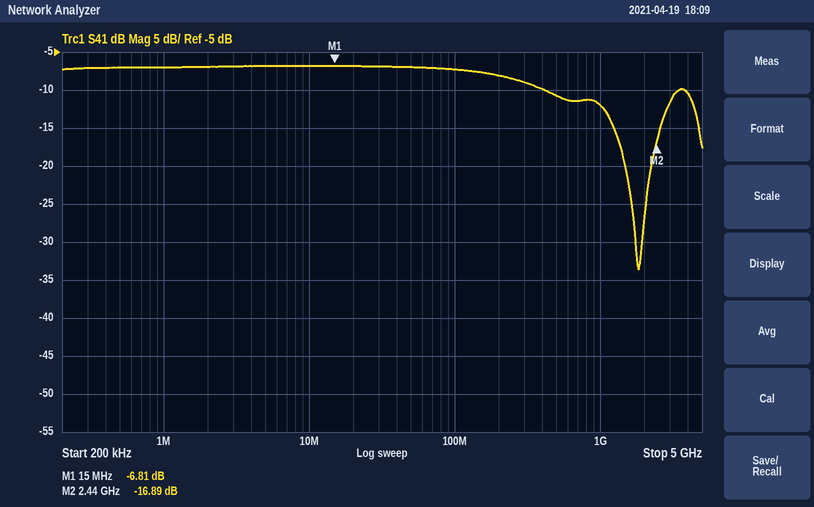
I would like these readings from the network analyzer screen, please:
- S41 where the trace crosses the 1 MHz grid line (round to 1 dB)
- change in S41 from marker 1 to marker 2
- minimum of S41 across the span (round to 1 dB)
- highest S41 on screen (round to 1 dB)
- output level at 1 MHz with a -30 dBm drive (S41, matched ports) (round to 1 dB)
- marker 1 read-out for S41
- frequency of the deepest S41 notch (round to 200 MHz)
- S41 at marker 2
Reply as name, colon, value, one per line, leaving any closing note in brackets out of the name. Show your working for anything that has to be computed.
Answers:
S41 where the trace crosses the 1 MHz grid line: -7 dB
change in S41 from marker 1 to marker 2: -16.89 − (-6.81) = -10.08 dB
minimum of S41 across the span: -34 dB
highest S41 on screen: -7 dB
output level at 1 MHz with a -30 dBm drive (S41, matched ports): -30 dBm + (-7 dB) = -37 dBm
marker 1 read-out for S41: -6.81 dB
frequency of the deepest S41 notch: 1.8 GHz
S41 at marker 2: -16.89 dB
